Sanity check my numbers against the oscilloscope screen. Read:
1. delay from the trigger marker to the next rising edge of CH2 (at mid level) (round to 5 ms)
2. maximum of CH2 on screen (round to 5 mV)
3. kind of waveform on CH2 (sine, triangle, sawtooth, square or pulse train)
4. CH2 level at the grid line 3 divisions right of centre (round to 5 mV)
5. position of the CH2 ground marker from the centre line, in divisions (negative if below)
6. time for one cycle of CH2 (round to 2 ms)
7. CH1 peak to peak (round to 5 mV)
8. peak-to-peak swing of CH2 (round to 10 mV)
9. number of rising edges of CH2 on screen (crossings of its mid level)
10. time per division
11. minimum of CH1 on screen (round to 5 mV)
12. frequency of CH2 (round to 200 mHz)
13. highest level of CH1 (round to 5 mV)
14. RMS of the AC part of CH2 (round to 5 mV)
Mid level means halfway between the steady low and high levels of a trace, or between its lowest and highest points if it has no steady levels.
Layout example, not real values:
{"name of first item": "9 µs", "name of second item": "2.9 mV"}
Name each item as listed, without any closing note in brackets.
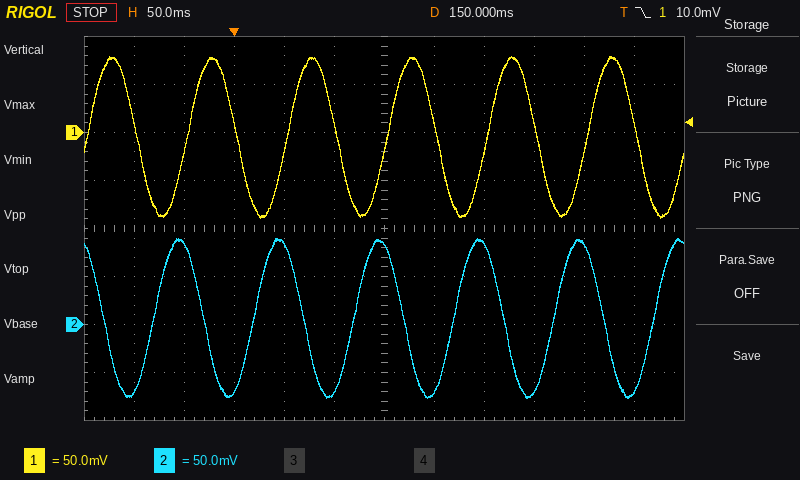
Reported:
{"delay from the trigger marker to the next rising edge of CH2 (at mid level)": "20 ms", "maximum of CH2 on screen": "90 mV", "kind of waveform on CH2": "sine", "CH2 level at the grid line 3 divisions right of centre": "-70 mV", "position of the CH2 ground marker from the centre line, in divisions": "-2.0 div", "time for one cycle of CH2": "100 ms", "CH1 peak to peak": "170 mV", "peak-to-peak swing of CH2": "170 mV", "number of rising edges of CH2 on screen": "6", "time per division": "50 ms", "minimum of CH1 on screen": "-90 mV", "frequency of CH2": "10.0 Hz", "highest level of CH1": "80 mV", "RMS of the AC part of CH2": "60 mV"}
